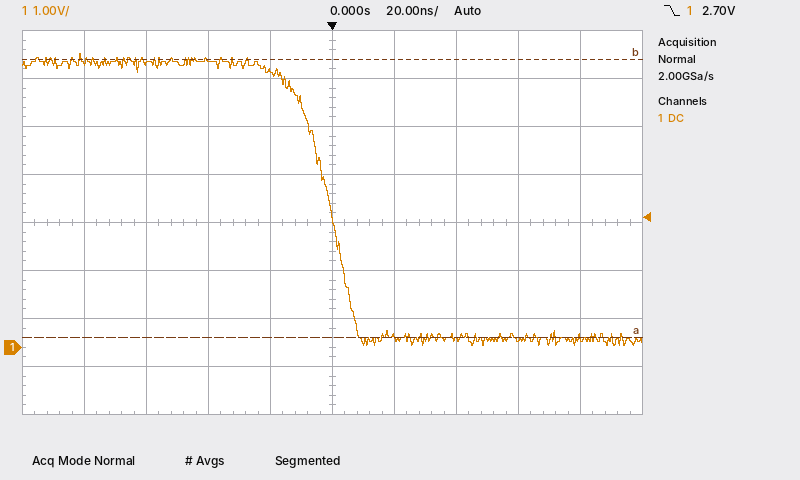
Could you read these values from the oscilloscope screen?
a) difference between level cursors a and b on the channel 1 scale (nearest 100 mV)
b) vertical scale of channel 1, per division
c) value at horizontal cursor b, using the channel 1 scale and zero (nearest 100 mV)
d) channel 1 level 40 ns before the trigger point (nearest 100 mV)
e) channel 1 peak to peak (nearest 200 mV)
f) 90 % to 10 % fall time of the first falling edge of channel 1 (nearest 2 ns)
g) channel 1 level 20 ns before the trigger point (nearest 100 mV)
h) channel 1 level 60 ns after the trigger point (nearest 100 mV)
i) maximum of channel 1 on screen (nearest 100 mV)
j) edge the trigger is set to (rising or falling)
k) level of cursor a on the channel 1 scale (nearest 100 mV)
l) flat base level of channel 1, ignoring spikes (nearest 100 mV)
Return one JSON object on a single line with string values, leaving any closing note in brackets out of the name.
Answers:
{"difference between level cursors a and b on the channel 1 scale": "5.8 V", "vertical scale of channel 1, per division": "1 V", "value at horizontal cursor b, using the channel 1 scale and zero": "6.0 V", "channel 1 level 40 ns before the trigger point": "6.0 V", "channel 1 peak to peak": "6.0 V", "90 % to 10 % fall time of the first falling edge of channel 1": "20 ns", "channel 1 level 20 ns before the trigger point": "5.7 V", "channel 1 level 60 ns after the trigger point": "200 mV", "maximum of channel 1 on screen": "6.1 V", "edge the trigger is set to": "falling", "level of cursor a on the channel 1 scale": "200 mV", "flat base level of channel 1, ignoring spikes": "200 mV"}
